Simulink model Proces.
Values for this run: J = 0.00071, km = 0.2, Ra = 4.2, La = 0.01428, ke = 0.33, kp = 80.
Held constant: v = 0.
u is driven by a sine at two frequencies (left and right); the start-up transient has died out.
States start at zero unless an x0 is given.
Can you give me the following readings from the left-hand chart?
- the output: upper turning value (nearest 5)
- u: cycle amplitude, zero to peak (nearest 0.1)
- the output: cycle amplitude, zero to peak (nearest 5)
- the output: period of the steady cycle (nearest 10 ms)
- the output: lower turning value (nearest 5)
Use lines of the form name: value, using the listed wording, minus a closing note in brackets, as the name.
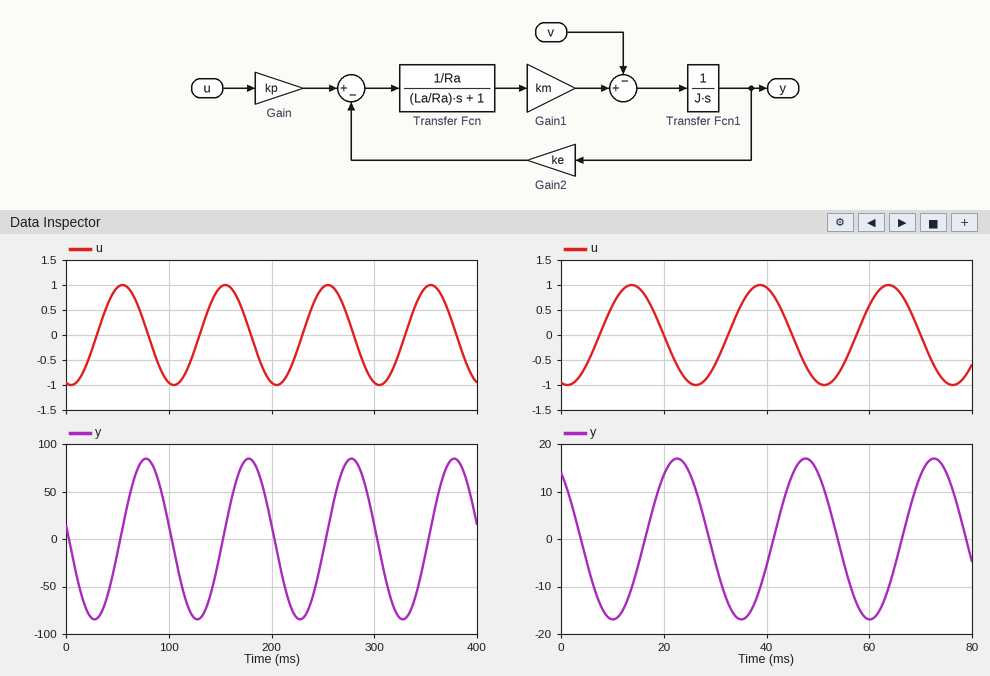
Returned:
the output: upper turning value: 85
u: cycle amplitude, zero to peak: 1.0
the output: cycle amplitude, zero to peak: 85
the output: period of the steady cycle: 100 ms
the output: lower turning value: -85
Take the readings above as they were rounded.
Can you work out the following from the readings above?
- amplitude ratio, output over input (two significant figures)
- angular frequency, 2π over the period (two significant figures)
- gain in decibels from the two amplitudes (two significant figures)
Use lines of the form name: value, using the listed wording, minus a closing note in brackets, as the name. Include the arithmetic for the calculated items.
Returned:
amplitude ratio, output over input: 85 / 1 = 85
angular frequency, 2π over the period: 2π / 100 = 0.063 rad/ms
gain in decibels from the two amplitudes: 20 log10(85 / 1) = 39 dB
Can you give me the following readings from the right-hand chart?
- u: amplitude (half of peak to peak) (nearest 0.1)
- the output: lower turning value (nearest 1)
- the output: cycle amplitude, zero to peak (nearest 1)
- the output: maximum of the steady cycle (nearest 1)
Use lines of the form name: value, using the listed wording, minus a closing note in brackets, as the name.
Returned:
u: amplitude (half of peak to peak): 1.0
the output: lower turning value: -17
the output: cycle amplitude, zero to peak: 17
the output: maximum of the steady cycle: 17
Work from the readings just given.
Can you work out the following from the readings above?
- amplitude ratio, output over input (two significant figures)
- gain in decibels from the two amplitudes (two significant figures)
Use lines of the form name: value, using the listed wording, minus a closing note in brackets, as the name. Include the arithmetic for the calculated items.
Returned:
amplitude ratio, output over input: 17 / 1 = 17
gain in decibels from the two amplitudes: 20 log10(17 / 1) = 25 dB
